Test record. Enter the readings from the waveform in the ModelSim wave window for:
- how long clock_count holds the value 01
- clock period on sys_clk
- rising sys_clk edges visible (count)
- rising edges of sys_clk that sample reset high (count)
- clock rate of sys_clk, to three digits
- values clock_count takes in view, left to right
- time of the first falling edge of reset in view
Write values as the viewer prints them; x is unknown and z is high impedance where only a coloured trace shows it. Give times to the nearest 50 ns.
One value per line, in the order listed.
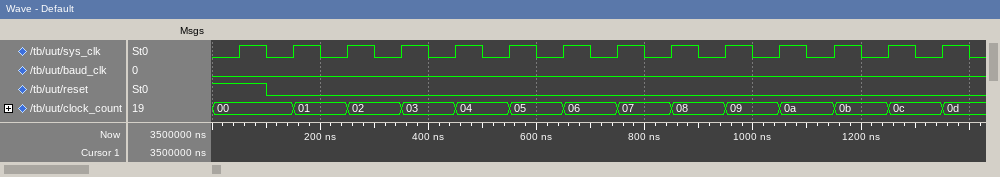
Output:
100 ns
100 ns
14
1
10.0 MHz
00, 01, 02, 03, 04, 05, 06, 07, 08, 09, 0a, 0b, 0c, 0d
100 ns
